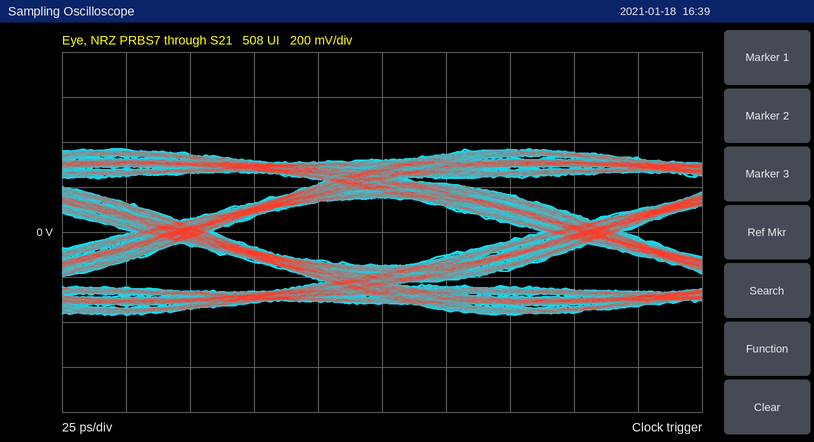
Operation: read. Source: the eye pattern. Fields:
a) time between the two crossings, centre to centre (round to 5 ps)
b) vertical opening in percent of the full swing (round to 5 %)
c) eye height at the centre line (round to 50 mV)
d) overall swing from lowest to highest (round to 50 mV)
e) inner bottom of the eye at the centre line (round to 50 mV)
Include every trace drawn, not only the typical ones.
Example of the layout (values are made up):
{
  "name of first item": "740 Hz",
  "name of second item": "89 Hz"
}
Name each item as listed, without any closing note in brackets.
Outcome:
{
  "time between the two crossings, centre to centre": "160 ps",
  "vertical opening in percent of the full swing": "40 %",
  "eye height at the centre line": "300 mV",
  "overall swing from lowest to highest": "750 mV",
  "inner bottom of the eye at the centre line": "-150 mV"
}
